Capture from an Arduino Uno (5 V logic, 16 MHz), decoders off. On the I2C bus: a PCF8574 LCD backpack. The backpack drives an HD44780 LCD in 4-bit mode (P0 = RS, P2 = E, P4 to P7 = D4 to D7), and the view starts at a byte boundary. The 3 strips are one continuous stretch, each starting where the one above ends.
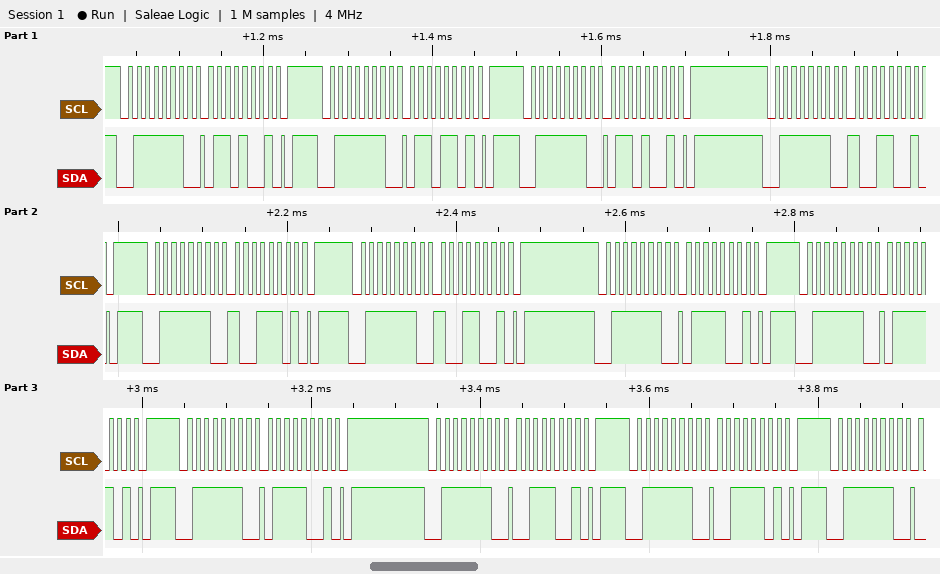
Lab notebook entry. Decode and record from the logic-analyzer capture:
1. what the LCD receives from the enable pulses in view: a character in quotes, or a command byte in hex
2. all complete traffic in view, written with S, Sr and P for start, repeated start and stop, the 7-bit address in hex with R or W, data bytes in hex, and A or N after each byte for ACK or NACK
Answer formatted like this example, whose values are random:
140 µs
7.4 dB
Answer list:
'i'
S 3FW A 69 A P S 3FW A 6D A P S 3FW A 69 A P S 3FW A 99 A P S 3FW A 9D A P S 3FW A 99 A P S 3FW A 79 A P S 3FW A 7D A P S 3FW A 79 A P S 3FW A 39 A P S 3FW A 3D A P S 3FW A
